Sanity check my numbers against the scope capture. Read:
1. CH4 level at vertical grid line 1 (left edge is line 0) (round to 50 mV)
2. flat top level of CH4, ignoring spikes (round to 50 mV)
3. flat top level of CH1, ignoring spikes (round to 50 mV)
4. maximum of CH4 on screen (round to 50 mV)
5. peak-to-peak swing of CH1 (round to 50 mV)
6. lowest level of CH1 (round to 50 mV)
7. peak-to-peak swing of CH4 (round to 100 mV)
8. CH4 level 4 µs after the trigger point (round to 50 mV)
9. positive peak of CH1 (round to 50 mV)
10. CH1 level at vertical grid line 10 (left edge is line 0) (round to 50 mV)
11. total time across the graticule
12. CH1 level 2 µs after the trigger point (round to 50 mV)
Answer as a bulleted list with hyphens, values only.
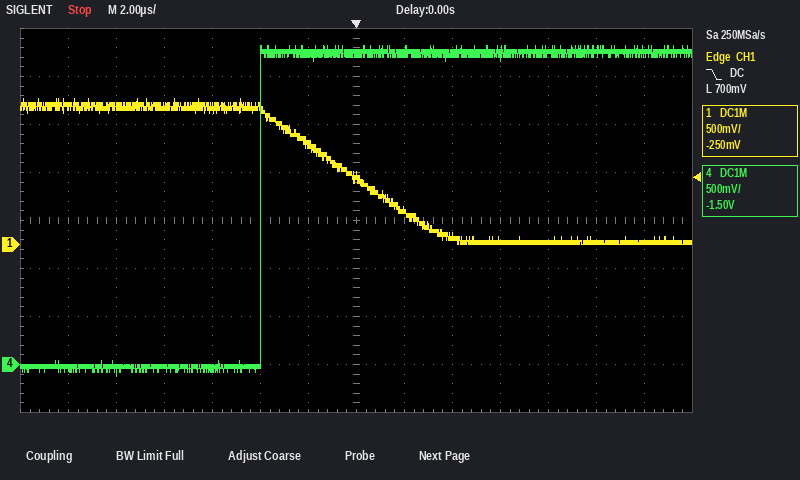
- -50 mV
- 3.25 V
- 1.45 V
- 3.30 V
- 1.50 V
- 0 mV
- 3.40 V
- 3.25 V
- 1.50 V
- 50 mV
- 28 µs
- 350 mV
